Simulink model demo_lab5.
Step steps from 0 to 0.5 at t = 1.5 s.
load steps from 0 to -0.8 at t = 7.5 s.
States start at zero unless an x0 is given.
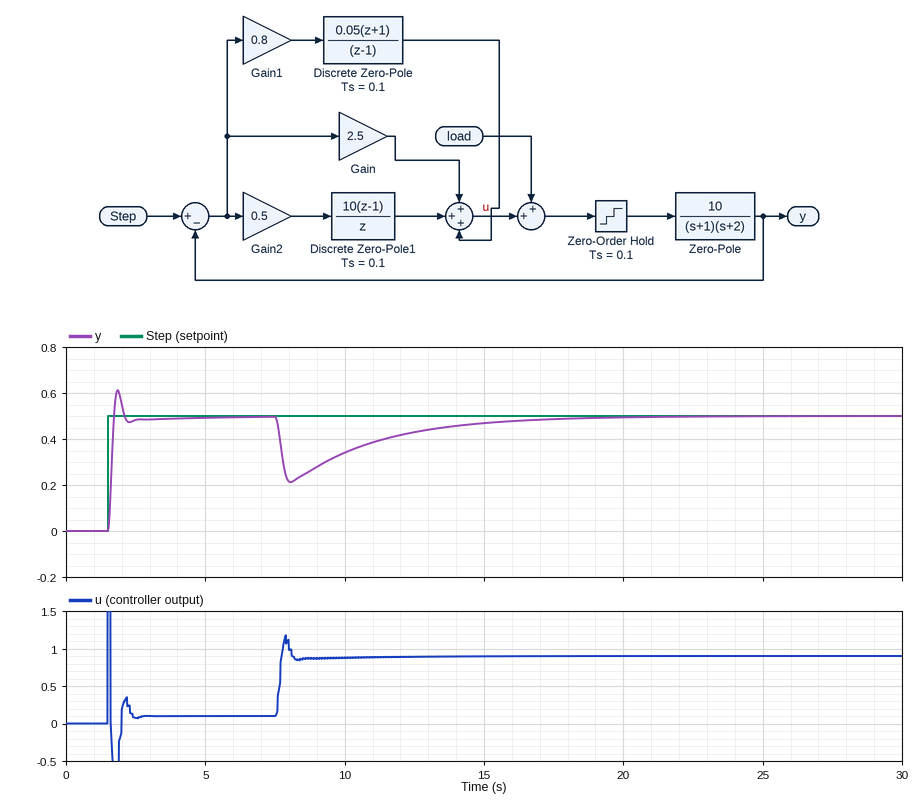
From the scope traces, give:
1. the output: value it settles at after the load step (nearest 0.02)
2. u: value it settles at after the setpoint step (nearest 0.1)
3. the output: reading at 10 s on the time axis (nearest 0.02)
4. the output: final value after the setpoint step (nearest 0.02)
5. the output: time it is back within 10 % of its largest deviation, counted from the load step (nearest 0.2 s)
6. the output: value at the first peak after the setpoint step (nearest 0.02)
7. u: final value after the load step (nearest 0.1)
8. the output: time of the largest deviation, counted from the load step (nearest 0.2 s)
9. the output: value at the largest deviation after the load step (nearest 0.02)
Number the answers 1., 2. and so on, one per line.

1. 0.50
2. 0.1
3. 0.34
4. 0.50
5. 7.8 s
6. 0.62
7. 0.9
8. 0.6 s
9. 0.22
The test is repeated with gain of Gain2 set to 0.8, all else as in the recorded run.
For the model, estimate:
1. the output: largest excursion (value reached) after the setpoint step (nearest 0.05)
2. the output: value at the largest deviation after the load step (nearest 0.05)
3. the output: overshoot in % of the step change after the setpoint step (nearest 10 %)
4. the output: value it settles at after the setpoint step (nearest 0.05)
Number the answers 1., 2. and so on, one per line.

1. 0.65
2. 0.25
3. 30 %
4. 0.50
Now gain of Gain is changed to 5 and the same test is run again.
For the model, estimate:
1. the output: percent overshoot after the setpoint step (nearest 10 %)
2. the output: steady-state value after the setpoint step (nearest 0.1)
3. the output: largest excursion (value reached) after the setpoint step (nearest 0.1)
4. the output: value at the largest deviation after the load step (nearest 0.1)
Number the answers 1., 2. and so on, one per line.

1. 60 %
2. 0.5
3. 0.8
4. 0.3
